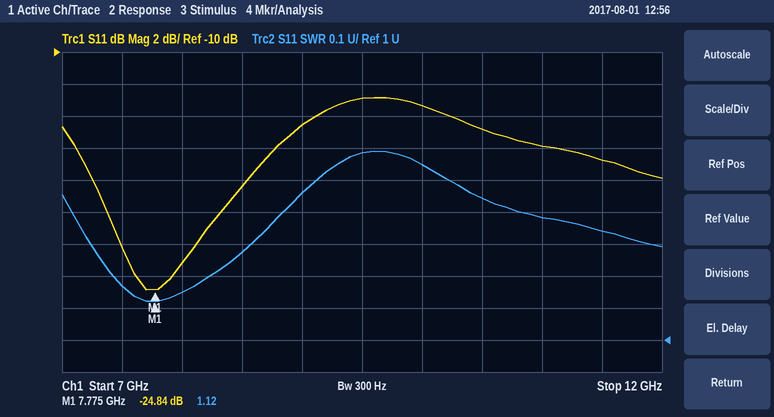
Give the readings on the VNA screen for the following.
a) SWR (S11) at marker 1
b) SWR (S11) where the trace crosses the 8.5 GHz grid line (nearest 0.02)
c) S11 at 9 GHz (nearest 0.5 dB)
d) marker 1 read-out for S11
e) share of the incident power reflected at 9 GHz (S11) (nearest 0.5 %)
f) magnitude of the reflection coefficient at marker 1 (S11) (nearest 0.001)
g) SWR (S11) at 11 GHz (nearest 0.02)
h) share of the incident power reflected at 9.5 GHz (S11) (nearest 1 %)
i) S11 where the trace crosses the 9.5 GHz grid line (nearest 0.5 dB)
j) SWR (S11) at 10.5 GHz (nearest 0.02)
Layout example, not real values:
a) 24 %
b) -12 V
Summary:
a) 1.12
b) 1.28
c) -14.5 dB
d) -24.84 dB
e) 3.5 %
f) 0.057
g) 1.38
h) 5 %
i) -13.0 dB
j) 1.44
